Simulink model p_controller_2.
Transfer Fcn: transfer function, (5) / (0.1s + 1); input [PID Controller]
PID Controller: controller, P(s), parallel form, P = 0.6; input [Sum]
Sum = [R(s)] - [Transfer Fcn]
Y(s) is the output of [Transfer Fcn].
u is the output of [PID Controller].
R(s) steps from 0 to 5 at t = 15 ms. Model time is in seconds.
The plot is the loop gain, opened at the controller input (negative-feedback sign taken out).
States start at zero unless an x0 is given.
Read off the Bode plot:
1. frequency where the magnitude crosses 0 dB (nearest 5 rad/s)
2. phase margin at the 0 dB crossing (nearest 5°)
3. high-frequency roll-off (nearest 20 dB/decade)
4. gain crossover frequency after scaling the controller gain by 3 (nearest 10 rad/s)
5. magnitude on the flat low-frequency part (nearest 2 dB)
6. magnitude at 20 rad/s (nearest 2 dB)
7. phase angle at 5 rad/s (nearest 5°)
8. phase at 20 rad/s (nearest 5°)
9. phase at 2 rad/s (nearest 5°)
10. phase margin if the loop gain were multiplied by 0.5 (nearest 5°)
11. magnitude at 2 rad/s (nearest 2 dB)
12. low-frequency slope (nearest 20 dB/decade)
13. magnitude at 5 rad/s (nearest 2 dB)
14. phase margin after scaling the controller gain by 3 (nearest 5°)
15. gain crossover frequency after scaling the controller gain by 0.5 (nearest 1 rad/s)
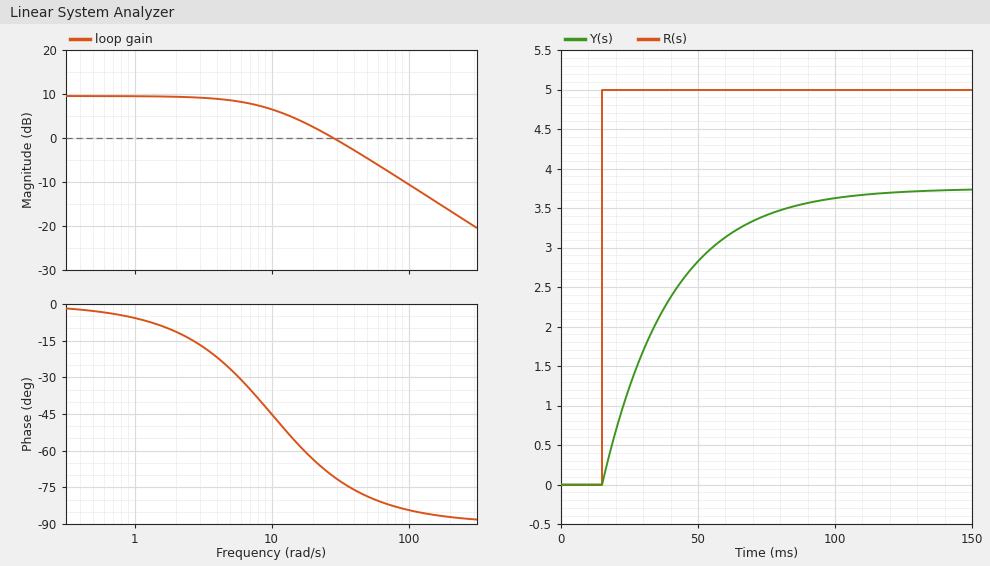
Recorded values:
30 rad/s
110°
-20 dB/decade
90 rad/s
10 dB
2 dB
-25°
-65°
-10°
130°
10 dB
0 dB/decade
8 dB
95°
11 rad/s
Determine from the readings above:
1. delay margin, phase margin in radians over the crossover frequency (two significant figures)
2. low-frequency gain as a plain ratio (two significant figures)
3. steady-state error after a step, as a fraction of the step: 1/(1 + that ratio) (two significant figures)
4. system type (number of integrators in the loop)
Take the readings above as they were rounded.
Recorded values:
0.064 s
3.2
0.24
0
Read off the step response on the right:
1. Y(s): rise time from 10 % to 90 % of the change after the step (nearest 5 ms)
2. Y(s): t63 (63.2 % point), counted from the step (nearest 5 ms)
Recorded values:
55 ms
25 ms
